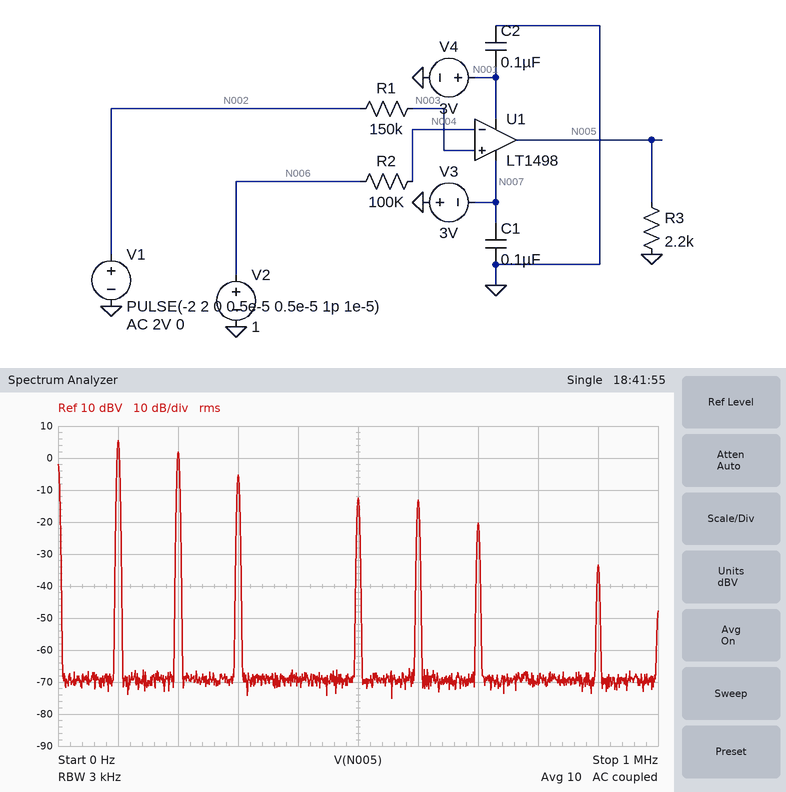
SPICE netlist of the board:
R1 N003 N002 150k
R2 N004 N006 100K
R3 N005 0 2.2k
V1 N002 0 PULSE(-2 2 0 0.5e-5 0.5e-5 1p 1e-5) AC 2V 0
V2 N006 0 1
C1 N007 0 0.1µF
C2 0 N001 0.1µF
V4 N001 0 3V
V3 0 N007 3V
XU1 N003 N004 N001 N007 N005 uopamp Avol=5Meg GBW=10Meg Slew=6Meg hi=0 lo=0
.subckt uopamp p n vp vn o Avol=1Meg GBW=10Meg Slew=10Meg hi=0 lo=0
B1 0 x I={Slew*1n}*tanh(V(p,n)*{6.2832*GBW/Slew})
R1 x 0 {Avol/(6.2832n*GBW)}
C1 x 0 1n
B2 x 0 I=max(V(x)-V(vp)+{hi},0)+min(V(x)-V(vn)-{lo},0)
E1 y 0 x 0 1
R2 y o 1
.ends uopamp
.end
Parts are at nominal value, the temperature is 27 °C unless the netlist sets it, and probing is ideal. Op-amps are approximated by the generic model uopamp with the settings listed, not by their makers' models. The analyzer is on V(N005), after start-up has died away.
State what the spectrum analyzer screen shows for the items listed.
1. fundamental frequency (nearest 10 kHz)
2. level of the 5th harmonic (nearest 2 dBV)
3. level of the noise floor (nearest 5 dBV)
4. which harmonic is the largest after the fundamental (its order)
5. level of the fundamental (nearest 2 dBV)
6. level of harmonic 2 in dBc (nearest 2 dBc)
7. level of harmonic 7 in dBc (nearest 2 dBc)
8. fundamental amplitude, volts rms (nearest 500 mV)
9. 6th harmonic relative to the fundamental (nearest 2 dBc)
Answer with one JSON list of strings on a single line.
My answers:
["100 kHz", "-12 dBV", "-70 dBV", "2", "6 dBV", "-4 dBc", "-26 dBc", "2.0 V", "-18 dBc"]
